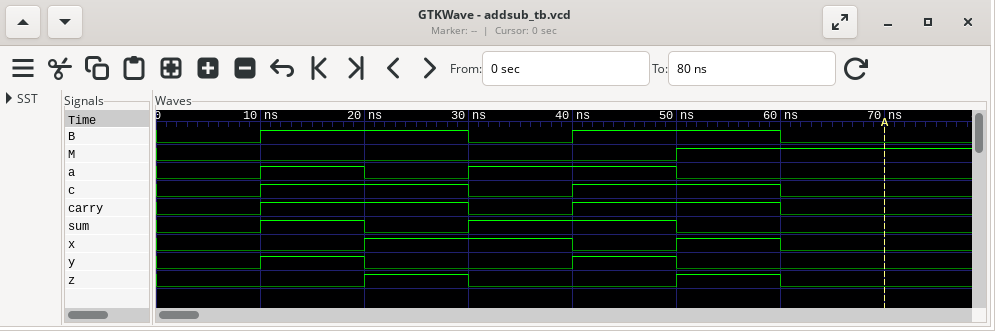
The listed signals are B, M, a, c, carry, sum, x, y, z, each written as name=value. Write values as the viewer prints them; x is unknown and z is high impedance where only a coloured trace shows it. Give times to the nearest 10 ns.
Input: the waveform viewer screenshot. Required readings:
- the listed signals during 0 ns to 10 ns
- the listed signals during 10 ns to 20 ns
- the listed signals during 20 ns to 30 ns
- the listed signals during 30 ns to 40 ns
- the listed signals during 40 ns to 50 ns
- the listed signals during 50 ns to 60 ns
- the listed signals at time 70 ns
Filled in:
B=0, M=0, a=0, c=0, carry=0, sum=0, x=0, y=0, z=0
B=1, M=0, a=1, c=1, carry=1, sum=1, x=0, y=1, z=0
B=1, M=0, a=0, c=1, carry=1, sum=0, x=1, y=0, z=1
B=0, M=0, a=1, c=0, carry=0, sum=1, x=1, y=0, z=0
B=1, M=0, a=1, c=1, carry=1, sum=1, x=0, y=1, z=0
B=1, M=1, a=0, c=1, carry=1, sum=0, x=1, y=0, z=1
B=0, M=1, a=0, c=0, carry=0, sum=0, x=0, y=0, z=0
